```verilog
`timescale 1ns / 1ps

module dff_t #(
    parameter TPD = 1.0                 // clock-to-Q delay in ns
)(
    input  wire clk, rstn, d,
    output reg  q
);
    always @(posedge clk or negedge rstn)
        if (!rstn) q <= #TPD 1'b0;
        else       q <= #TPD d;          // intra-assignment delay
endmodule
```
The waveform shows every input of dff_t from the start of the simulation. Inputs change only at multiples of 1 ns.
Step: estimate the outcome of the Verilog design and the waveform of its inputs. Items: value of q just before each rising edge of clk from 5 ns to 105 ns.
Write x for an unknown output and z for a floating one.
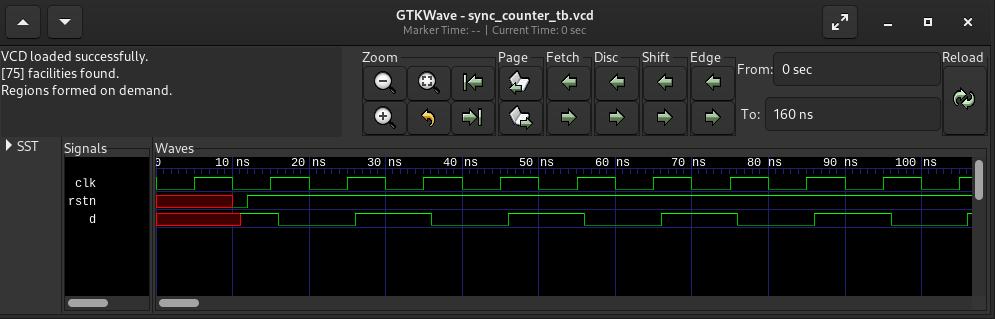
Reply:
x 0 1 0 1 0 1 0 1 0 1
